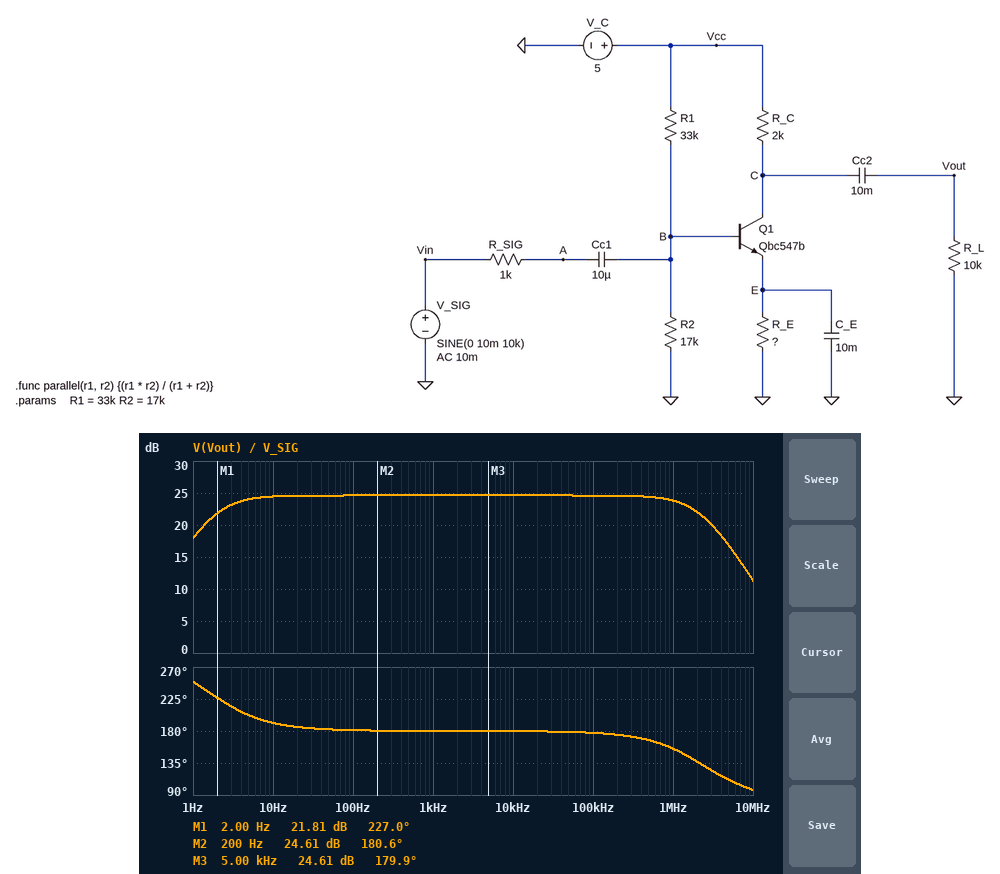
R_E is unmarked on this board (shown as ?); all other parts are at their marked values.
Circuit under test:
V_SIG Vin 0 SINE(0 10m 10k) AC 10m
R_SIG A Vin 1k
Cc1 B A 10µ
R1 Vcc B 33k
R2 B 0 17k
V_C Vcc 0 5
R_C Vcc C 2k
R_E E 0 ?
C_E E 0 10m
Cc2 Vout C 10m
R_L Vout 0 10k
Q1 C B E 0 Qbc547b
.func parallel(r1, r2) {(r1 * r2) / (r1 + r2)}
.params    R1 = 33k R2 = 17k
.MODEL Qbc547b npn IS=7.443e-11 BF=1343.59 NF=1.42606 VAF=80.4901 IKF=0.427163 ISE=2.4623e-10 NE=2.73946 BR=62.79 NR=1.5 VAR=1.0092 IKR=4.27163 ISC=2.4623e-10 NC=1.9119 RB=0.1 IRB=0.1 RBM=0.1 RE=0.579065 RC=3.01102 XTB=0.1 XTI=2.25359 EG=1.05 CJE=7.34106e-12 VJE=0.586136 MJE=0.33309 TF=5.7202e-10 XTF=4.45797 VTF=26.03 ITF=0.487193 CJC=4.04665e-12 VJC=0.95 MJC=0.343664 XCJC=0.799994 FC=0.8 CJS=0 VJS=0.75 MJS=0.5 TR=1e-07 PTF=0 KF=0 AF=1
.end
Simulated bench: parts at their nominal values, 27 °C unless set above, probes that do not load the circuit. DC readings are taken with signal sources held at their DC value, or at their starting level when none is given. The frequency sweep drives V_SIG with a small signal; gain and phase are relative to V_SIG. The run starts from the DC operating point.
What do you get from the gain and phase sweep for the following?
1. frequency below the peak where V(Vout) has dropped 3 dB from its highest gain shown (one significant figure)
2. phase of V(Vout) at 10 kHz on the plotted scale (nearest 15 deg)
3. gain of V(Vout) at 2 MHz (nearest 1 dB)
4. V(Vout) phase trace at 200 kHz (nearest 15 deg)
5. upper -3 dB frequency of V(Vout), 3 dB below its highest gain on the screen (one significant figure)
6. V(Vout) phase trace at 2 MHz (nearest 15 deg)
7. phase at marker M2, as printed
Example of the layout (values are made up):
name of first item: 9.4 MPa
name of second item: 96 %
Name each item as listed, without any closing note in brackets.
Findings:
frequency below the peak where V(Vout) has dropped 3 dB from its highest gain shown: 2 Hz
phase of V(Vout) at 10 kHz on the plotted scale: 180 deg
gain of V(Vout) at 2 MHz: 22 dB
V(Vout) phase trace at 200 kHz: 180 deg
upper -3 dB frequency of V(Vout), 3 dB below its highest gain on the screen: 2 MHz
V(Vout) phase trace at 2 MHz: 135 deg
phase at marker M2, as printed: 180.6 deg
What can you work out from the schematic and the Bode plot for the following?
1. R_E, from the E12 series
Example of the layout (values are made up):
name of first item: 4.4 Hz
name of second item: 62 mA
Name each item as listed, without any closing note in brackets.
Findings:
R_E, from the E12 series: 2.2 kΩ
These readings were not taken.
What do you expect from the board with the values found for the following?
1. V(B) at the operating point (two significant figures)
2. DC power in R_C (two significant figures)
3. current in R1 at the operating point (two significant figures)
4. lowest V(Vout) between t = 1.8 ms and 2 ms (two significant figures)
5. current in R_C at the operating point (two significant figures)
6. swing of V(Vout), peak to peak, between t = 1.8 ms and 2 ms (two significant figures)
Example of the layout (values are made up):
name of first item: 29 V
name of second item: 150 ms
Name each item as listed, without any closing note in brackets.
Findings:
V(B) at the operating point: 1.7 V
DC power in R_C: 460 µW
current in R1 at the operating point: 100 µA
lowest V(Vout) between t = 1.8 ms and 2 ms: -190 mV
current in R_C at the operating point: 480 µA
swing of V(Vout), peak to peak, between t = 1.8 ms and 2 ms: 340 mV
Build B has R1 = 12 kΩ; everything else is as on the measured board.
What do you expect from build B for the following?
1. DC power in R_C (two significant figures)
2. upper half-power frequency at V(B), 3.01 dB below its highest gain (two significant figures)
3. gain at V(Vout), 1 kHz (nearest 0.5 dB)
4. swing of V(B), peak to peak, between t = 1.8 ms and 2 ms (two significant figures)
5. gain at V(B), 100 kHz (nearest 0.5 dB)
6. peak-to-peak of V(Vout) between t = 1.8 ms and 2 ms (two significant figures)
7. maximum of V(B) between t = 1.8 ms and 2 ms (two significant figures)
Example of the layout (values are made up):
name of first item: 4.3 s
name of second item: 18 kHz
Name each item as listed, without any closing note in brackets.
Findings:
DC power in R_C: 2.1 mW
upper half-power frequency at V(B), 3.01 dB below its highest gain: 1.0 MHz
gain at V(Vout), 1 kHz: 30.0 dB
swing of V(B), peak to peak, between t = 1.8 ms and 2 ms: 16 mV
gain at V(B), 100 kHz: -2.0 dB
peak-to-peak of V(Vout) between t = 1.8 ms and 2 ms: 620 mV
maximum of V(B) between t = 1.8 ms and 2 ms: 2.9 V
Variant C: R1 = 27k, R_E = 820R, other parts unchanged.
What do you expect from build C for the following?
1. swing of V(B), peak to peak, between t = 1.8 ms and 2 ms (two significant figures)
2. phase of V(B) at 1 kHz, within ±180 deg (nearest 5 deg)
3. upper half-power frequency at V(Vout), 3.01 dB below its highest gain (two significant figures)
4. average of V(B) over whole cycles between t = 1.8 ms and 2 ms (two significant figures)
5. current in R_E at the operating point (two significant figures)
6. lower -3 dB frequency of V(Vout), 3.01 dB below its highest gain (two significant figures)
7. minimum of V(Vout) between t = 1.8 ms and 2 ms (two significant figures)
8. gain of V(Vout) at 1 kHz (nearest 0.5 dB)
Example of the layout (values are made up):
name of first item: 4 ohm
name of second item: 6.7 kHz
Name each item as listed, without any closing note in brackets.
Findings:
swing of V(B), peak to peak, between t = 1.8 ms and 2 ms: 16 mV
phase of V(B) at 1 kHz, within ±180 deg: 0 deg
upper half-power frequency at V(Vout), 3.01 dB below its highest gain: 780 kHz
average of V(B) over whole cycles between t = 1.8 ms and 2 ms: 1.9 V
current in R_E at the operating point: 1.5 mA
lower -3 dB frequency of V(Vout), 3.01 dB below its highest gain: 3.1 Hz
minimum of V(Vout) between t = 1.8 ms and 2 ms: -460 mV
gain of V(Vout) at 1 kHz: 33.0 dB
